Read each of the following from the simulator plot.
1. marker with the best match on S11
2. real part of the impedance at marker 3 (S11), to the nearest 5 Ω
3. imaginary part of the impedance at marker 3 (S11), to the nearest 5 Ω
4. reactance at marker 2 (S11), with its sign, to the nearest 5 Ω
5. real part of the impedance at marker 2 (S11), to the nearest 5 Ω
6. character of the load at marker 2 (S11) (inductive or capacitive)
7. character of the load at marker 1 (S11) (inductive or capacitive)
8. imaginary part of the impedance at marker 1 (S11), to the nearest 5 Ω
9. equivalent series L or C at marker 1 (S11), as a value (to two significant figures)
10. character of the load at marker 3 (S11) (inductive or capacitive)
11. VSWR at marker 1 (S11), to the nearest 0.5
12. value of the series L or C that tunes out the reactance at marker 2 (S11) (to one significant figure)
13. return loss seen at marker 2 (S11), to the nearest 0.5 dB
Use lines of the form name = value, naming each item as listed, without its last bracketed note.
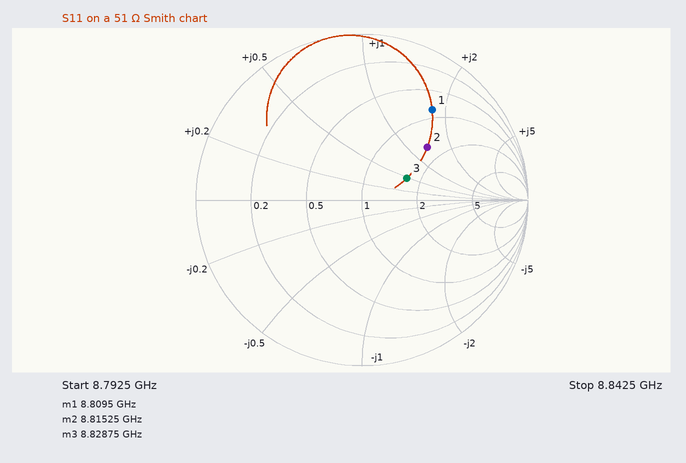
marker with the best match on S11 = marker 3
real part of the impedance at marker 3 (S11), to the nearest 5 Ω = 85 Ω
imaginary part of the impedance at marker 3 (S11), to the nearest 5 Ω = +25 Ω
reactance at marker 2 (S11), with its sign, to the nearest 5 Ω = +70 Ω
real part of the impedance at marker 2 (S11), to the nearest 5 Ω = 80 Ω
character of the load at marker 2 (S11) = inductive
character of the load at marker 1 (S11) = inductive
imaginary part of the impedance at marker 1 (S11), to the nearest 5 Ω = +90 Ω
equivalent series L or C at marker 1 (S11), as a value = 1.6 nH
character of the load at marker 3 (S11) = inductive
VSWR at marker 1 (S11), to the nearest 0.5 = 5.5
value of the series L or C that tunes out the reactance at marker 2 (S11) = 300 fF
return loss seen at marker 2 (S11), to the nearest 0.5 dB = 6.0 dB
